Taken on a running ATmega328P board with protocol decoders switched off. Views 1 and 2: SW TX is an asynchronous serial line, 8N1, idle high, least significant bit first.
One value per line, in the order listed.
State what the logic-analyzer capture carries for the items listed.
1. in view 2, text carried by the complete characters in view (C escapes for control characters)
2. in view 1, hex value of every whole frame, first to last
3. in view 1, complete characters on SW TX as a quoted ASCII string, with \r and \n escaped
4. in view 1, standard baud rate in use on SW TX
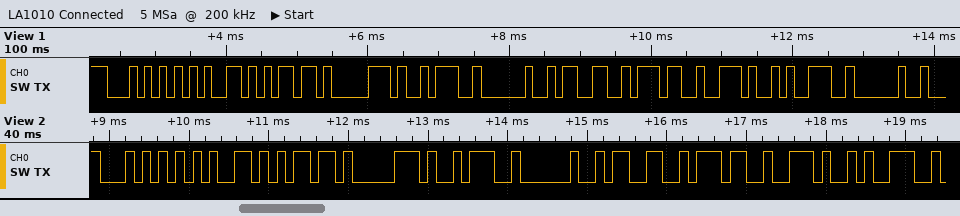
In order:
"Temp: 37.9"
0x54 0x65 0x6D 0x70 0x3A 0x20 0x33 0x37 0x2E 0x39 0x20
"Temp: 37.9 "
9600 baud
